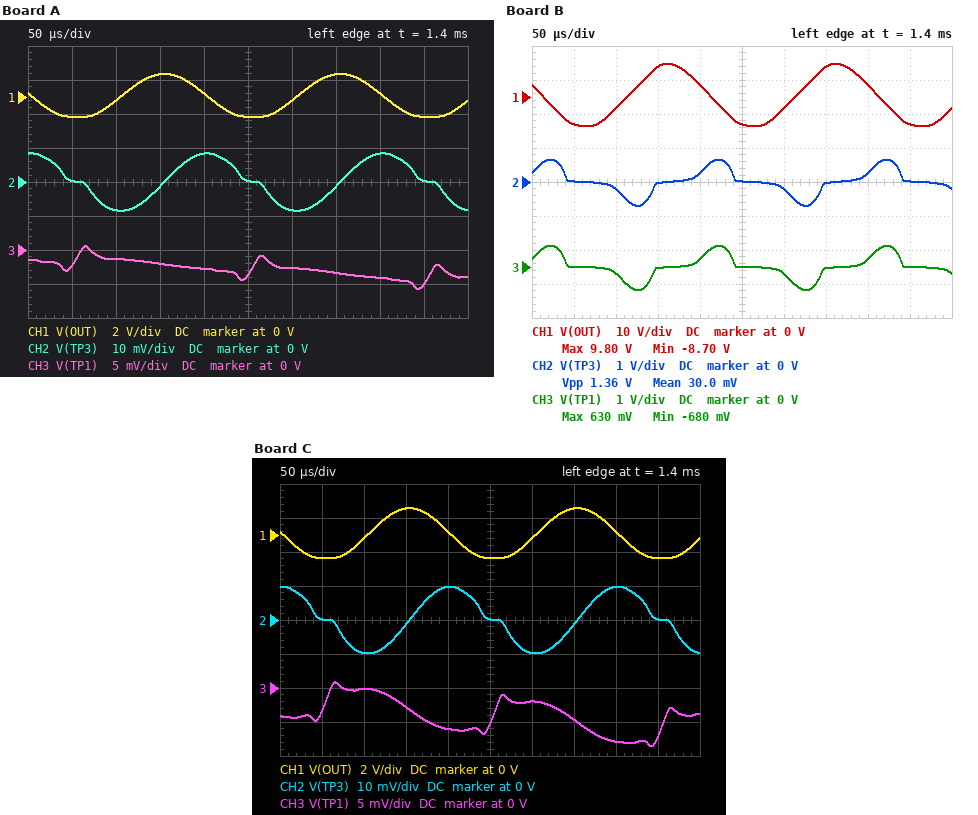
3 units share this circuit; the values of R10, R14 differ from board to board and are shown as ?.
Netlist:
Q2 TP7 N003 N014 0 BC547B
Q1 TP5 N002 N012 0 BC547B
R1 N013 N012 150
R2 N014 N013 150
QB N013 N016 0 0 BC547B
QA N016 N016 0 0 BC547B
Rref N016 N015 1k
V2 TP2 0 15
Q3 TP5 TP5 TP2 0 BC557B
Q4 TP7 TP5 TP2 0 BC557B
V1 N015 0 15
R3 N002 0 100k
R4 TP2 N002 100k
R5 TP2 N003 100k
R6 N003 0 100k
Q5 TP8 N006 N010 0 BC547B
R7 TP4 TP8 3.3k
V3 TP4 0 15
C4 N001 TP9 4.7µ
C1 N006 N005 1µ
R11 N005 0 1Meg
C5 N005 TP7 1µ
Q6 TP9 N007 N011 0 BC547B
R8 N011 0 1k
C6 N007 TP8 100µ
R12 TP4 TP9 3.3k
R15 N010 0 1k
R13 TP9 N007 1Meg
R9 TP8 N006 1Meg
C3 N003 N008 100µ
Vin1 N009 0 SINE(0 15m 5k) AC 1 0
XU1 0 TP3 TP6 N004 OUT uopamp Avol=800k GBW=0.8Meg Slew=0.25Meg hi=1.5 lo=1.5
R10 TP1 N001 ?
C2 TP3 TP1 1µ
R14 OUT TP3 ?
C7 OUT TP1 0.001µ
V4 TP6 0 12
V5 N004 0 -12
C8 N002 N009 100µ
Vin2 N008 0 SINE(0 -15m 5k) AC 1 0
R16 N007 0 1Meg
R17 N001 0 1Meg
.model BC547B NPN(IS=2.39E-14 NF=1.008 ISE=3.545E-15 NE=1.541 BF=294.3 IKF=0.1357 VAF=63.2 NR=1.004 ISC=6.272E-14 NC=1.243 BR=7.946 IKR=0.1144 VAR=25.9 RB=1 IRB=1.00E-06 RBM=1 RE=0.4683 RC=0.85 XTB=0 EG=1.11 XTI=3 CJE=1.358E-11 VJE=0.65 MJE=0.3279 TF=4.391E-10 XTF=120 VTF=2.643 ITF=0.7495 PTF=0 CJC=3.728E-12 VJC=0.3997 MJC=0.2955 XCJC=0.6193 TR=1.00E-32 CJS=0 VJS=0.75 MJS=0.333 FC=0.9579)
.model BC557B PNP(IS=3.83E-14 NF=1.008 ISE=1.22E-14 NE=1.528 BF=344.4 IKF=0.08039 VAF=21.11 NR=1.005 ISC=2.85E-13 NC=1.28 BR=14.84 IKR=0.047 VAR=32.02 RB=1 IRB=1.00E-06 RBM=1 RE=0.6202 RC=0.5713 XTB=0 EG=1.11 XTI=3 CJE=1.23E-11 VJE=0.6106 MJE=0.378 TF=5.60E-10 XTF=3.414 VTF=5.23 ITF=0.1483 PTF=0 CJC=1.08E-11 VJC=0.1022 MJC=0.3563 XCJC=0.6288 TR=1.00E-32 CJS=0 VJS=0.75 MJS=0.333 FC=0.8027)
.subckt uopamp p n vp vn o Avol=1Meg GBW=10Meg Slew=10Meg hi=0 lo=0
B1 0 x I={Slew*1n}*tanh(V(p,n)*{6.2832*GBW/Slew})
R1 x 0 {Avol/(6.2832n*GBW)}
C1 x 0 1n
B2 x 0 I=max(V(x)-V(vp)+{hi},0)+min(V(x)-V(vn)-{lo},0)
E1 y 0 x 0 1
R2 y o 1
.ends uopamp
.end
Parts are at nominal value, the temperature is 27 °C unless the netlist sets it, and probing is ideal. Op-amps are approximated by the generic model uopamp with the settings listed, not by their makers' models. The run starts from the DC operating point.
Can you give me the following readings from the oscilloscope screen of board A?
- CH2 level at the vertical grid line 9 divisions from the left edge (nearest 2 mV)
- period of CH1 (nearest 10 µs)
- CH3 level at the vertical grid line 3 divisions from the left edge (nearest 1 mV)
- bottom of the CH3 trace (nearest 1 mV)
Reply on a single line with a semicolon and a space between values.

0 V; 200 µs; -2 mV; -6 mV
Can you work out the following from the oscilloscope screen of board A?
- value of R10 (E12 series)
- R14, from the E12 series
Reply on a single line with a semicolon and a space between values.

18 kΩ; 4.7 kΩ
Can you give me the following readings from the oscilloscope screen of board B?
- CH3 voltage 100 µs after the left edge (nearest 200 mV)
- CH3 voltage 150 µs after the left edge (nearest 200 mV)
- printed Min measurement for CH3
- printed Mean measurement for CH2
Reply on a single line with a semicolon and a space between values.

-200 mV; 0 V; -680 mV; 30.0 mV
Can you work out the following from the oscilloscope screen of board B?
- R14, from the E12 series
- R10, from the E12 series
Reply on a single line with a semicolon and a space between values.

10 kΩ; 2.7 kΩ
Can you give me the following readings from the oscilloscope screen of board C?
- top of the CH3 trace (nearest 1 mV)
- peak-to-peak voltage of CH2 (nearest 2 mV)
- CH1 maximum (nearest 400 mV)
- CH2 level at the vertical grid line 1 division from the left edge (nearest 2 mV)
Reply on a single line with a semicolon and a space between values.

1 mV; 20 mV; 1.6 V; 0 V
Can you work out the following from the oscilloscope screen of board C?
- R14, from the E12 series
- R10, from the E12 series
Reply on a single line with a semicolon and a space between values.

3.9 kΩ; 12 kΩ
